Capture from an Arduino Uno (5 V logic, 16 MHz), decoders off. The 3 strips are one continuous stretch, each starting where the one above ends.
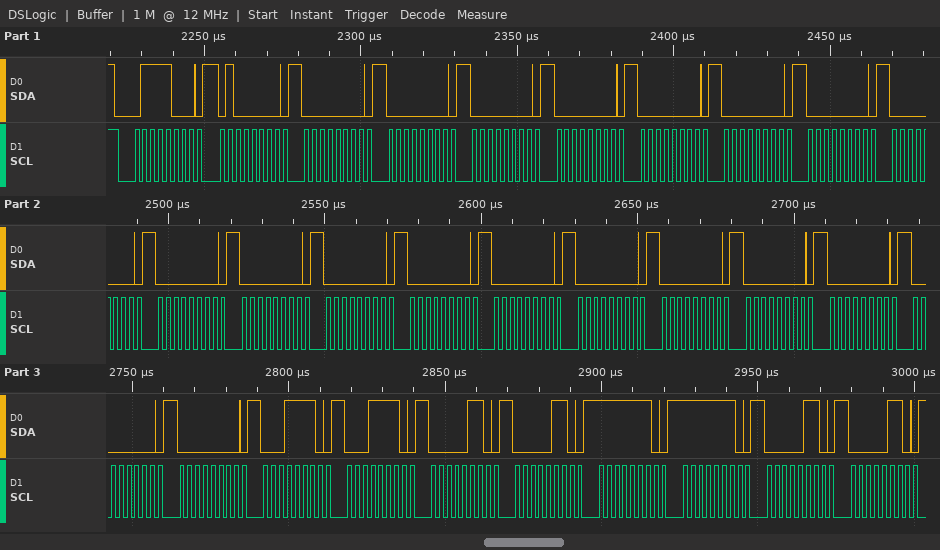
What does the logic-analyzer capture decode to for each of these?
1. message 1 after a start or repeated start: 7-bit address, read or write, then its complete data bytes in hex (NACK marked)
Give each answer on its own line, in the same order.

0x3C write: 40 00 00 00 00 00 00 00 00 00 00 00 00 00 00 00 00 00 00 00 1E 1E 06 06 FE FE 06 06
